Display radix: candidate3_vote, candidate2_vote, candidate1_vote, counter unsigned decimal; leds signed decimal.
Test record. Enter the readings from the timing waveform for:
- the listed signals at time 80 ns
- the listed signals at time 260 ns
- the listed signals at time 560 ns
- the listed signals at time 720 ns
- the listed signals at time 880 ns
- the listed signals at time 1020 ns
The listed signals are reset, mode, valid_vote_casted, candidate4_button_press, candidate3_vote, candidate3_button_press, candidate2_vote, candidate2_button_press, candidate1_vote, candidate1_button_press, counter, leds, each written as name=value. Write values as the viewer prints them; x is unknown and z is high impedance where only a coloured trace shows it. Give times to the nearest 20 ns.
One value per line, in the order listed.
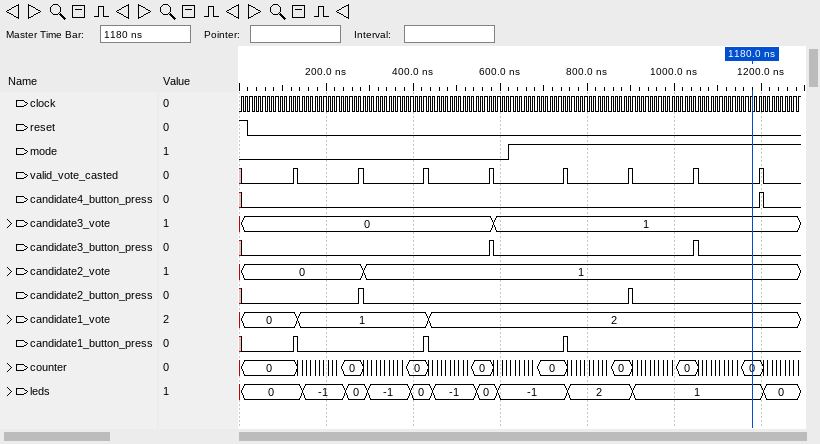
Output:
reset=0, mode=0, valid_vote_casted=0, candidate4_button_press=0, candidate3_vote=0, candidate3_button_press=0, candidate2_vote=0, candidate2_button_press=0, candidate1_vote=0, candidate1_button_press=0, counter=0, leds=0
reset=0, mode=0, valid_vote_casted=0, candidate4_button_press=0, candidate3_vote=0, candidate3_button_press=0, candidate2_vote=0, candidate2_button_press=0, candidate1_vote=1, candidate1_button_press=0, counter=0, leds=0
reset=0, mode=0, valid_vote_casted=0, candidate4_button_press=0, candidate3_vote=0, candidate3_button_press=0, candidate2_vote=1, candidate2_button_press=0, candidate1_vote=2, candidate1_button_press=0, counter=0, leds=0
reset=0, mode=1, valid_vote_casted=0, candidate4_button_press=0, candidate3_vote=1, candidate3_button_press=0, candidate2_vote=1, candidate2_button_press=0, candidate1_vote=2, candidate1_button_press=0, counter=0, leds=-1
reset=0, mode=1, valid_vote_casted=0, candidate4_button_press=0, candidate3_vote=1, candidate3_button_press=0, candidate2_vote=1, candidate2_button_press=0, candidate1_vote=2, candidate1_button_press=0, counter=0, leds=2
reset=0, mode=1, valid_vote_casted=0, candidate4_button_press=0, candidate3_vote=1, candidate3_button_press=0, candidate2_vote=1, candidate2_button_press=0, candidate1_vote=2, candidate1_button_press=0, counter=0, leds=1
